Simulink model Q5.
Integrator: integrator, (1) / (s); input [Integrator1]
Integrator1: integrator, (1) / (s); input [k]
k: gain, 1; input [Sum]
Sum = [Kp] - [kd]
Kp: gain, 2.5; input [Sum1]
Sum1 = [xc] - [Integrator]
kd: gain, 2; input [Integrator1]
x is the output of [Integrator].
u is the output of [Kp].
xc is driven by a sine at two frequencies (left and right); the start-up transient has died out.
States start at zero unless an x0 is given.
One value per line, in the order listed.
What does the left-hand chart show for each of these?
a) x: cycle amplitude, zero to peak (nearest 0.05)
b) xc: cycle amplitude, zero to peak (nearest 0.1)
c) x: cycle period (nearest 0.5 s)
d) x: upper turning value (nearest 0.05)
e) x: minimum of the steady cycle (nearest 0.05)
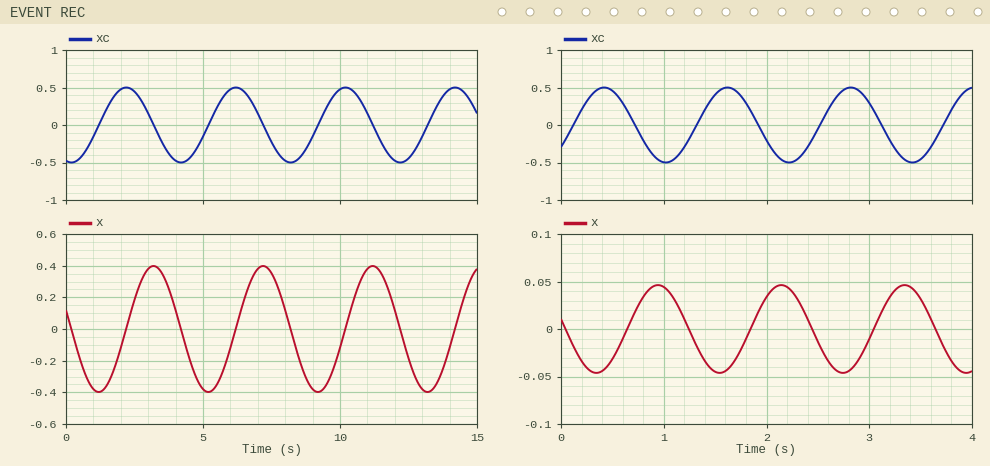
0.40
0.5
4.0 s
0.40
-0.40
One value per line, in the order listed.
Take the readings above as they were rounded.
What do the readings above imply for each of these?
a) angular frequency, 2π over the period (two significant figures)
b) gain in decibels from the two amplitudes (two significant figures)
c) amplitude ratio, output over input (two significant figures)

1.6 rad/s
-1.9 dB
0.80
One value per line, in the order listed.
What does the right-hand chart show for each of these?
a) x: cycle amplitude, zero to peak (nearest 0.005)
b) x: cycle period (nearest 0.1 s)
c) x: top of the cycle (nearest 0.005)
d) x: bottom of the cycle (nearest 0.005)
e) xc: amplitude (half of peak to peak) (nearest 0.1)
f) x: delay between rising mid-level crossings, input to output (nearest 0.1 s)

0.045
1.2 s
0.045
-0.045
0.5
0.5 s
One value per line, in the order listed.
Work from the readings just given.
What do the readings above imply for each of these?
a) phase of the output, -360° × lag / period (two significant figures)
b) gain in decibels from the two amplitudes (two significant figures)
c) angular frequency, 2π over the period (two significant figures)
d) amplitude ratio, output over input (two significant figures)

-150°
-21 dB
5.2 rad/s
0.090
